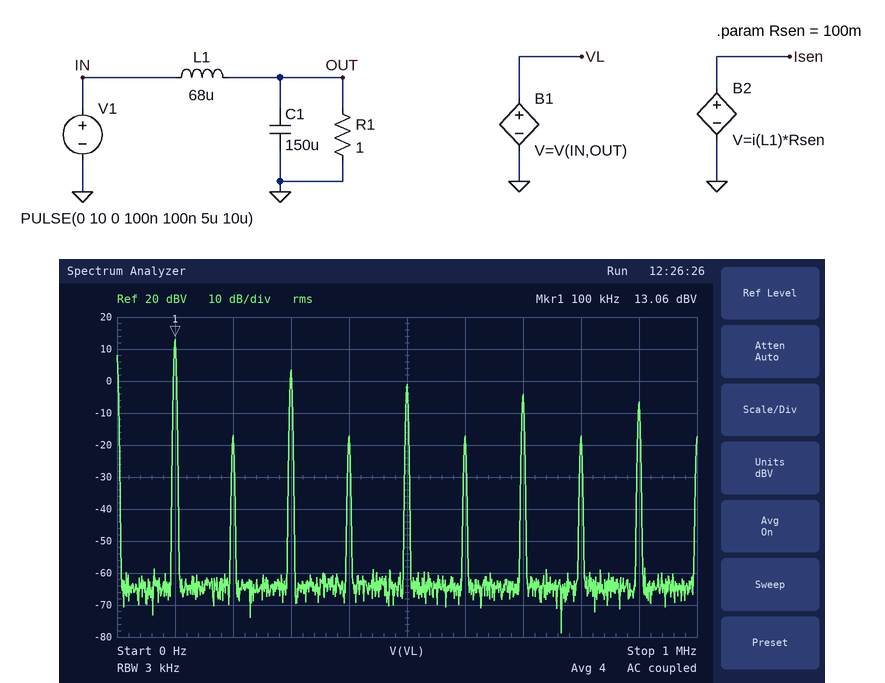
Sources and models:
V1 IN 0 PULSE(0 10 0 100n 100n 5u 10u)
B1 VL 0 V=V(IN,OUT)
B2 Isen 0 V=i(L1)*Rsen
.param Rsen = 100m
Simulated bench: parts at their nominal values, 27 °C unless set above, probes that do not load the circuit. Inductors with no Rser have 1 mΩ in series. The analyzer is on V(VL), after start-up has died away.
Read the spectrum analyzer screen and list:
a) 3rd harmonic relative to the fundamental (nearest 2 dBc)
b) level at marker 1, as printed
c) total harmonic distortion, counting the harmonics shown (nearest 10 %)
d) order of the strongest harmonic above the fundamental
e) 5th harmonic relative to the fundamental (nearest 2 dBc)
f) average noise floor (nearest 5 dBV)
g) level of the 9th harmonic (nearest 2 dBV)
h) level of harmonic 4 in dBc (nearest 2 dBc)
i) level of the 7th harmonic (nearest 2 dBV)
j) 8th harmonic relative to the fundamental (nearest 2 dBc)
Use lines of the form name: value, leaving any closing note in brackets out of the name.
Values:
3rd harmonic relative to the fundamental: -10 dBc
level at marker 1, as printed: 13.06 dBV
total harmonic distortion, counting the harmonics shown: 40 %
order of the strongest harmonic above the fundamental: 3
5th harmonic relative to the fundamental: -14 dBc
average noise floor: -65 dBV
level of the 9th harmonic: -6 dBV
level of harmonic 4 in dBc: -30 dBc
level of the 7th harmonic: -4 dBV
8th harmonic relative to the fundamental: -30 dBc
